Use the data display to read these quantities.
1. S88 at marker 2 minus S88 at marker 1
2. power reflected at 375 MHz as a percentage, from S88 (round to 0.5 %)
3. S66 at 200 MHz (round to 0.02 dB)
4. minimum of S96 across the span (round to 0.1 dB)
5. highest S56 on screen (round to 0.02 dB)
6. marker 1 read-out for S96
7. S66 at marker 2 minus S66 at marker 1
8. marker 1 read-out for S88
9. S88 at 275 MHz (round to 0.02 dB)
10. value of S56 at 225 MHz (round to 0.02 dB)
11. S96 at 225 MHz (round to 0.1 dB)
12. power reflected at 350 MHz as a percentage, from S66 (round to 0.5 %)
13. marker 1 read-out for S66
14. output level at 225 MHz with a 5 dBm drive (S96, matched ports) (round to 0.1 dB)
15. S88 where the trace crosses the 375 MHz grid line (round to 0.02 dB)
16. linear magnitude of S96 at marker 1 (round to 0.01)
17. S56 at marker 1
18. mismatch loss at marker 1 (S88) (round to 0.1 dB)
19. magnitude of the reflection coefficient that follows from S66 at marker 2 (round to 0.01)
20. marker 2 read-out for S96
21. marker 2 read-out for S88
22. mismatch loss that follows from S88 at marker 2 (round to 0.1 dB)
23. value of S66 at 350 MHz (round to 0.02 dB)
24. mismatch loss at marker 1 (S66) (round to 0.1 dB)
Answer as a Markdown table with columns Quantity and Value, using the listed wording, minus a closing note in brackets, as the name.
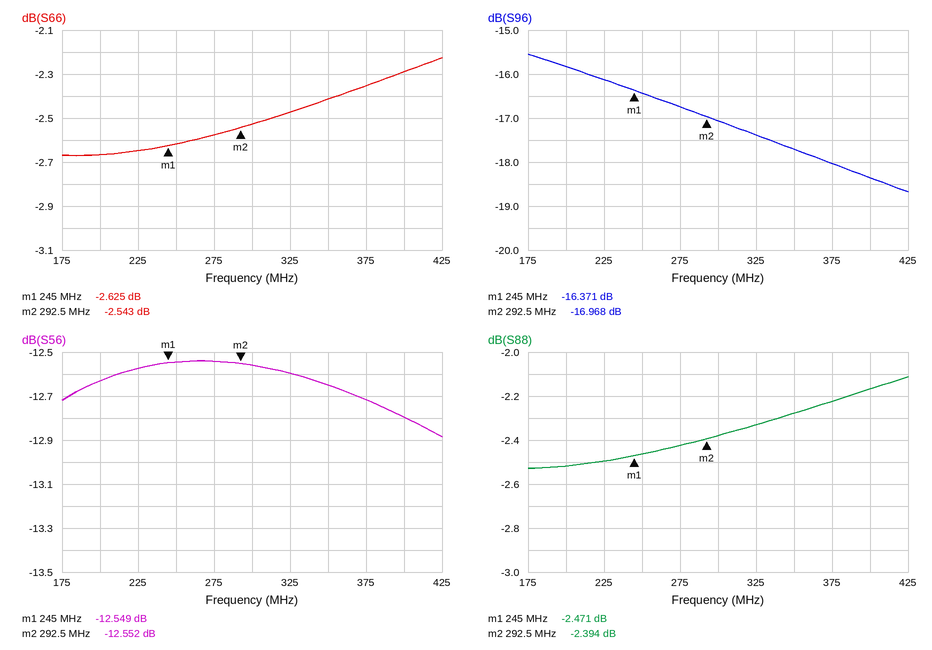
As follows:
| Quantity | Value |
|---|---|
| S88 at marker 2 minus S88 at marker 1 | 0.077 dB |
| power reflected at 375 MHz as a percentage, from S88 | 60.0 % |
| S66 at 200 MHz | -2.66 dB |
| minimum of S96 across the span | -18.7 dB |
| highest S56 on screen | -12.54 dB |
| marker 1 read-out for S96 | -16.371 dB |
| S66 at marker 2 minus S66 at marker 1 | 0.082 dB |
| marker 1 read-out for S88 | -2.471 dB |
| S88 at 275 MHz | -2.42 dB |
| value of S56 at 225 MHz | -12.58 dB |
| S96 at 225 MHz | -16.1 dB |
| power reflected at 350 MHz as a percentage, from S66 | 57.5 % |
| marker 1 read-out for S66 | -2.625 dB |
| output level at 225 MHz with a 5 dBm drive (S96, matched ports) | -11.1 dBm |
| S88 where the trace crosses the 375 MHz grid line | -2.22 dB |
| linear magnitude of S96 at marker 1 | 0.15 |
| S56 at marker 1 | -12.549 dB |
| mismatch loss at marker 1 (S88) | 3.6 dB |
| magnitude of the reflection coefficient that follows from S66 at marker 2 | 0.75 |
| marker 2 read-out for S96 | -16.968 dB |
| marker 2 read-out for S88 | -2.394 dB |
| mismatch loss that follows from S88 at marker 2 | 3.7 dB |
| value of S66 at 350 MHz | -2.42 dB |
| mismatch loss at marker 1 (S66) | 3.4 dB |
